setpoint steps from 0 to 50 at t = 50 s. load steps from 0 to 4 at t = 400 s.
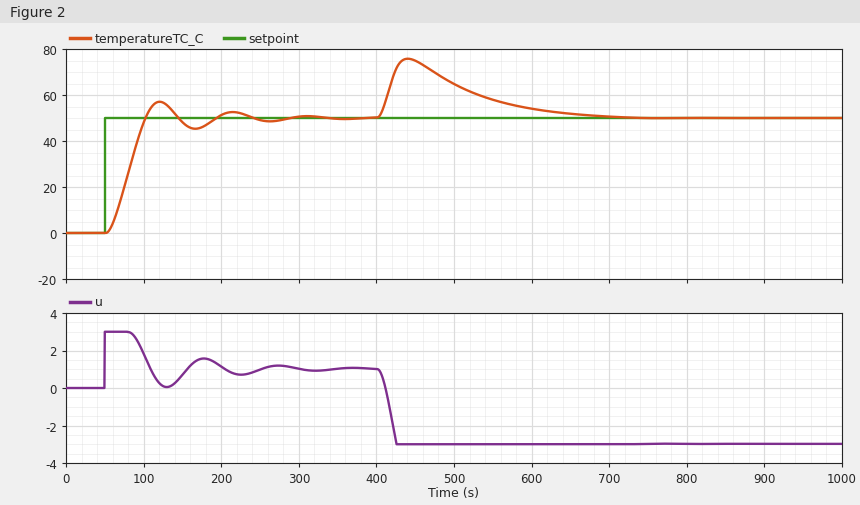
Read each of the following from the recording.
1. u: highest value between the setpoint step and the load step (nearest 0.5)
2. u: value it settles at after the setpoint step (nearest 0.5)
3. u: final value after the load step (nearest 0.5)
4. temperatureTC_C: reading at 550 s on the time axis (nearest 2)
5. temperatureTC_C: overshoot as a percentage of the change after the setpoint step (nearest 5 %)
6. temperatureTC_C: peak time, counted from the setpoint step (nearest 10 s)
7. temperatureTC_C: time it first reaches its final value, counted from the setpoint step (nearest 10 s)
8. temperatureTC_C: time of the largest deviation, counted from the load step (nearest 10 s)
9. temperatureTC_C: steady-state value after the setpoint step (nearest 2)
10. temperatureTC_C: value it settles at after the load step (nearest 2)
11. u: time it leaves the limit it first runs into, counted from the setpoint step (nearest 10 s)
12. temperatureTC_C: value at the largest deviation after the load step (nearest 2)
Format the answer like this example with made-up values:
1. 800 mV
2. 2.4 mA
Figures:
1. 3.0
2. 1.0
3. -3.0
4. 58
5. 15 %
6. 70 s
7. 50 s
8. 40 s
9. 50
10. 50
11. 30 s
12. 76
